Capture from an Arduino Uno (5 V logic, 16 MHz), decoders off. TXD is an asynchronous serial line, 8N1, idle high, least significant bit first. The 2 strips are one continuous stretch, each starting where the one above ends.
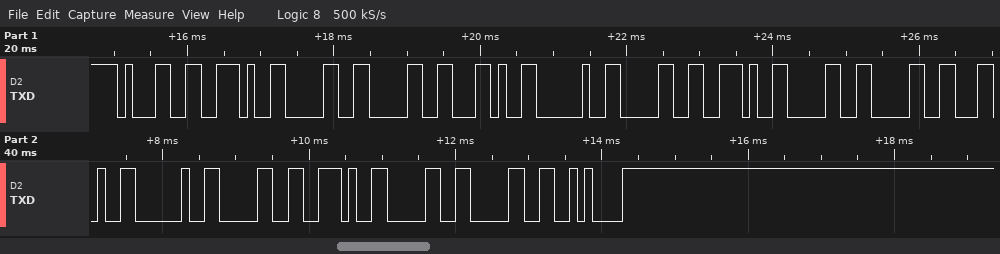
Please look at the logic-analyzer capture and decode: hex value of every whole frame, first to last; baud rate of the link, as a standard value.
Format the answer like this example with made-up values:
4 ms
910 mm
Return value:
0x31 0x2E 0x30 0x30 0x2C 0x20 0x30 0x2E 0x30 0x30 0x2C 0x20 0x30 0x2E 0x30 0x30 0x0A
9600 baud
